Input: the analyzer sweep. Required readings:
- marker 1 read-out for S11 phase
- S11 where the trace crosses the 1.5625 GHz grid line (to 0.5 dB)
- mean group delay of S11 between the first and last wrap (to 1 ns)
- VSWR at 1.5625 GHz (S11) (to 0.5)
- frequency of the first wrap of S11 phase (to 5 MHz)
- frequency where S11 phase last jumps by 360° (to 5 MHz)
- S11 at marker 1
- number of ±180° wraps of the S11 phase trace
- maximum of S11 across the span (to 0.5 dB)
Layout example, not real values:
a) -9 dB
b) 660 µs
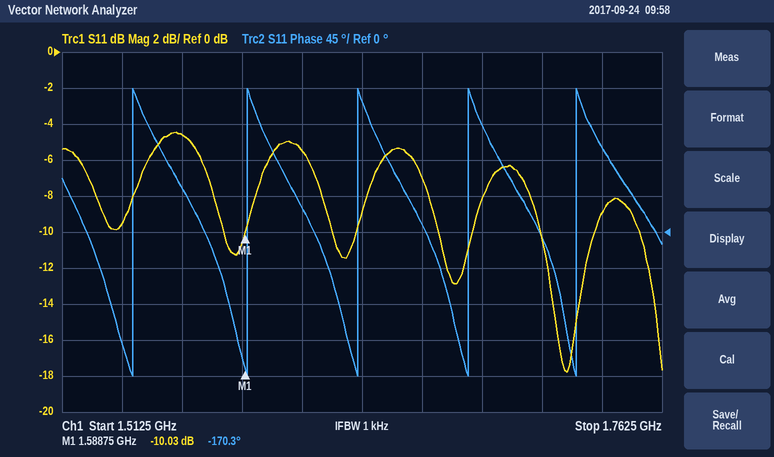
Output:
a) -170.3°
b) -4.5 dB
c) 22 ns
d) 4.0
e) 1.540 GHz
f) 1.725 GHz
g) -10.03 dB
h) 5
i) -4.5 dB
